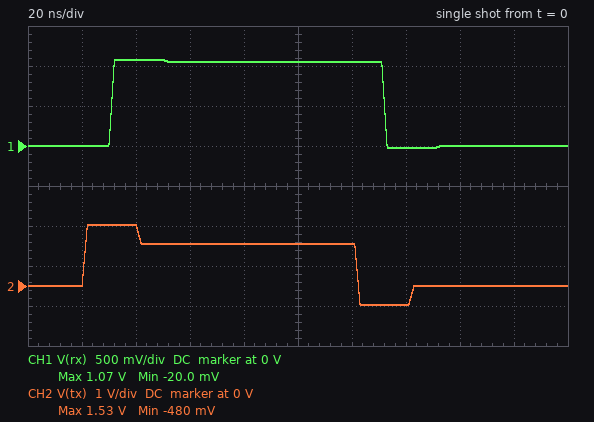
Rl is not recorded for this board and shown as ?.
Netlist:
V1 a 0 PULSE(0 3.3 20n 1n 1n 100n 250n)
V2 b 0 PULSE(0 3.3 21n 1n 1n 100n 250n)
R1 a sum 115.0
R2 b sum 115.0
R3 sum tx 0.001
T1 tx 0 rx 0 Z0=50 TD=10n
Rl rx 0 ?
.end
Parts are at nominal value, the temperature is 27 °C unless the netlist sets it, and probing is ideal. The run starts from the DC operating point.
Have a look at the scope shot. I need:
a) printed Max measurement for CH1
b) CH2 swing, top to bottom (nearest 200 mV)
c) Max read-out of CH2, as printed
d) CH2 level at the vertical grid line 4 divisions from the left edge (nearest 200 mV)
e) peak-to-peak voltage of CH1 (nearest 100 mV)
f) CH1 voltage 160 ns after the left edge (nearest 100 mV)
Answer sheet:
1.07 V
2.0 V
1.53 V
1.0 V
1.1 V
0 V
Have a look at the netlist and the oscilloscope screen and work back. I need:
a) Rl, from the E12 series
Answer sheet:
27 Ω
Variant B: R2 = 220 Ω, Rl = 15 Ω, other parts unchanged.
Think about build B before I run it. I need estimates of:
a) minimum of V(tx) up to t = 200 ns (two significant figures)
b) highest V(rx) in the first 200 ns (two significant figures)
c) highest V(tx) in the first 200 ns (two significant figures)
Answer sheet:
-770 mV
610 mV
1.3 V
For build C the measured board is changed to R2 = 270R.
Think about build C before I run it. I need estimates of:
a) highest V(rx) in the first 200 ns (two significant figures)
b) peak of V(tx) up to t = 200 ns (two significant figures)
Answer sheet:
890 mV
1.3 V
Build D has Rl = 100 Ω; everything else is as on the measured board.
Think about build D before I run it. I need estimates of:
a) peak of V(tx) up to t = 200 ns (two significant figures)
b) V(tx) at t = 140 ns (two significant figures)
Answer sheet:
2.1 V
560 mV
